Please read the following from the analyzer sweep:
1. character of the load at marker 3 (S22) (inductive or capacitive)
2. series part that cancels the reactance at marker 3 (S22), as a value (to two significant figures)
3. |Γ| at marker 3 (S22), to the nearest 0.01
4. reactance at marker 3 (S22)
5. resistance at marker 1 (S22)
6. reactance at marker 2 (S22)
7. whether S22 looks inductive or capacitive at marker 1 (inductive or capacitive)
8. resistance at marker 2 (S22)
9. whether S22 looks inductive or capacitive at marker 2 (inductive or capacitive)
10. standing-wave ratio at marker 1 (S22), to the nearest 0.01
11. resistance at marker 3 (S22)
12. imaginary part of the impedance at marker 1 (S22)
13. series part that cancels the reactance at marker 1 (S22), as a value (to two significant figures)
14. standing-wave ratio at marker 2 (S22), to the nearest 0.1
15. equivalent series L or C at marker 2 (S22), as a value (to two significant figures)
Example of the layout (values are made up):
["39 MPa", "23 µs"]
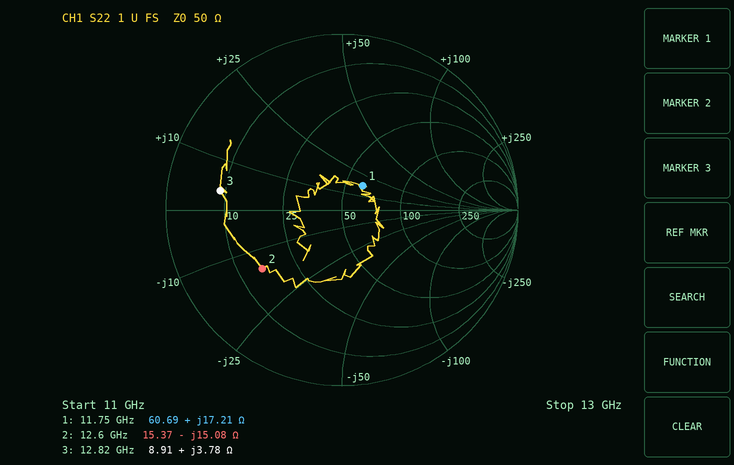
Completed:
["inductive", "3.3 pF", "0.70", "+3.78 Ω", "60.69 Ω", "-15.08 Ω", "inductive", "15.37 Ω", "capacitive", "1.44", "8.91 Ω", "+17.21 Ω", "790 fF", "3.6", "840 fF"]
